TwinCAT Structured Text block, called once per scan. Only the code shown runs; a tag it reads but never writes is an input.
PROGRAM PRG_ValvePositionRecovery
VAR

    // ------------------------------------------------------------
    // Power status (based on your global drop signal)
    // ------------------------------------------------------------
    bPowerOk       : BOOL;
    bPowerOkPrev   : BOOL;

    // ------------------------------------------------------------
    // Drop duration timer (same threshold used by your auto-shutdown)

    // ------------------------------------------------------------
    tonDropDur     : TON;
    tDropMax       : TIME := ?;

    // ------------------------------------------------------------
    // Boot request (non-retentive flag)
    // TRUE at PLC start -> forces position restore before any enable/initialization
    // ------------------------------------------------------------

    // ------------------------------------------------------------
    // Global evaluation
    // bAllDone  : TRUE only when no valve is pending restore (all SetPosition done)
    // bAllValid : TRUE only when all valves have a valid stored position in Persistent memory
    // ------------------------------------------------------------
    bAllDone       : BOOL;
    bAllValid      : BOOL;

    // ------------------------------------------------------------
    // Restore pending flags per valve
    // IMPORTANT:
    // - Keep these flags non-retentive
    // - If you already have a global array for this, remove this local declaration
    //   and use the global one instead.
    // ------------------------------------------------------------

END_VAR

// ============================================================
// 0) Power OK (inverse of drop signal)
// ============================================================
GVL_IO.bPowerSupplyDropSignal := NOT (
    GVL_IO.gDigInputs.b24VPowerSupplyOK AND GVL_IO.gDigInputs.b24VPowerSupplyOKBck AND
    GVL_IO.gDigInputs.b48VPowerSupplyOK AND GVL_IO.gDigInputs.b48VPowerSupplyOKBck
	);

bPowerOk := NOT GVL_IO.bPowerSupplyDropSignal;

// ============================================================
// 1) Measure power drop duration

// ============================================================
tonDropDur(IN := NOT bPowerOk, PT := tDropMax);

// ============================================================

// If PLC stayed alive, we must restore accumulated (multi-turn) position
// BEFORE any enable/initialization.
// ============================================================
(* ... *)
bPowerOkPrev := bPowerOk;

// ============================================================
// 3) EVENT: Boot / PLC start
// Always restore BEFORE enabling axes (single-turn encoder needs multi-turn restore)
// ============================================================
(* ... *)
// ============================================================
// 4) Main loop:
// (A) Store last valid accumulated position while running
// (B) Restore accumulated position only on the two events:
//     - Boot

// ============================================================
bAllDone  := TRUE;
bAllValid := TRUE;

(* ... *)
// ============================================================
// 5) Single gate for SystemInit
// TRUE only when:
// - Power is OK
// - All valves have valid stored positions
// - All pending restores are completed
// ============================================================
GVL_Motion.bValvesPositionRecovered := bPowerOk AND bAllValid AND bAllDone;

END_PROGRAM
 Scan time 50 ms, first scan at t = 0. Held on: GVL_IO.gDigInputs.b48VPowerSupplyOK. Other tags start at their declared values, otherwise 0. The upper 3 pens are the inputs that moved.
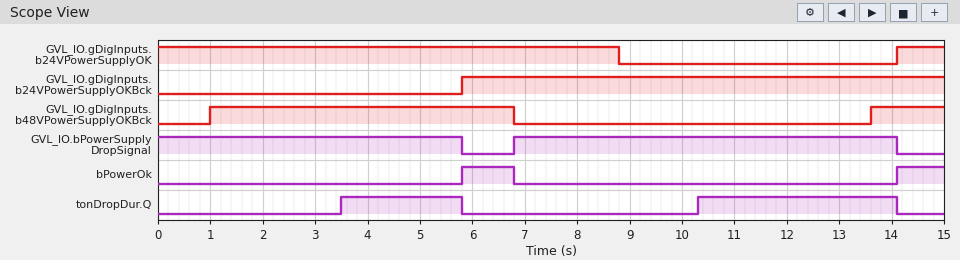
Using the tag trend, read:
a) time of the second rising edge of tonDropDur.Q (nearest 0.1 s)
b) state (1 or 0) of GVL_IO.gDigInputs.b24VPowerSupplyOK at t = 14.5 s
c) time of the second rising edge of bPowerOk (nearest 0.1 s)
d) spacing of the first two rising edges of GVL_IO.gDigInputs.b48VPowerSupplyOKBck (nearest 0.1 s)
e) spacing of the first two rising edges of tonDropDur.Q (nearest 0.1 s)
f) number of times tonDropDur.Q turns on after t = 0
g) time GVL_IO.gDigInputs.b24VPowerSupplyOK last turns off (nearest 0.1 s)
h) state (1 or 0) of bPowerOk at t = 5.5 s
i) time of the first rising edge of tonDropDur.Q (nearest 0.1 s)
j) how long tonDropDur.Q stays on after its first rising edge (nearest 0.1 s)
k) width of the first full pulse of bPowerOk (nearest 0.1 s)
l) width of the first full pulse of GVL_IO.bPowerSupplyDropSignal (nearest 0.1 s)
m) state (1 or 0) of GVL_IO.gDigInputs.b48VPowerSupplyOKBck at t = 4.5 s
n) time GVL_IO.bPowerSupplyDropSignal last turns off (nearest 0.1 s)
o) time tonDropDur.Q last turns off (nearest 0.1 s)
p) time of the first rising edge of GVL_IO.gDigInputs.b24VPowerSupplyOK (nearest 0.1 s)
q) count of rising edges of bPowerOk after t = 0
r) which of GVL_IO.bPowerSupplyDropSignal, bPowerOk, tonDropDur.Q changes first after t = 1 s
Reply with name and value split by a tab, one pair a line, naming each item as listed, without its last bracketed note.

time of the second rising edge of tonDropDur.Q	10.3 s
state (1 or 0) of GVL_IO.gDigInputs.b24VPowerSupplyOK at t = 14.5 s	1
time of the second rising edge of bPowerOk	14.1 s
spacing of the first two rising edges of GVL_IO.gDigInputs.b48VPowerSupplyOKBck	12.6 s
spacing of the first two rising edges of tonDropDur.Q	6.8 s
number of times tonDropDur.Q turns on after t = 0	2
time GVL_IO.gDigInputs.b24VPowerSupplyOK last turns off	8.8 s
state (1 or 0) of bPowerOk at t = 5.5 s	0
time of the first rising edge of tonDropDur.Q	3.5 s
how long tonDropDur.Q stays on after its first rising edge	2.3 s
width of the first full pulse of bPowerOk	1.0 s
width of the first full pulse of GVL_IO.bPowerSupplyDropSignal	7.3 s
state (1 or 0) of GVL_IO.gDigInputs.b48VPowerSupplyOKBck at t = 4.5 s	1
time GVL_IO.bPowerSupplyDropSignal last turns off	14.1 s
time tonDropDur.Q last turns off	14.1 s
time of the first rising edge of GVL_IO.gDigInputs.b24VPowerSupplyOK	14.1 s
count of rising edges of bPowerOk after t = 0	2
which of GVL_IO.bPowerSupplyDropSignal, bPowerOk, tonDropDur.Q changes first after t = 1 s	tonDropDur.Q
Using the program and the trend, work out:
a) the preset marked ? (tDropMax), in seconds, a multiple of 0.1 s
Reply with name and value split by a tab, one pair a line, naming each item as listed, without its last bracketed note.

the preset marked ? (tDropMax), in seconds, a multiple of 0.1 s	3.5 s
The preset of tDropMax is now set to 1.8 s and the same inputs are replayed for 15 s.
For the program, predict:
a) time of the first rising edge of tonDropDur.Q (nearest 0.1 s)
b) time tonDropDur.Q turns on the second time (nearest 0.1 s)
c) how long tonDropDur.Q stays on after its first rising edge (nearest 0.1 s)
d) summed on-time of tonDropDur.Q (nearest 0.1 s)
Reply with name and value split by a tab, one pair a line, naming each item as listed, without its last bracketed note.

time of the first rising edge of tonDropDur.Q	1.8 s
time tonDropDur.Q turns on the second time	8.6 s
how long tonDropDur.Q stays on after its first rising edge	4.0 s
summed on-time of tonDropDur.Q	9.5 s
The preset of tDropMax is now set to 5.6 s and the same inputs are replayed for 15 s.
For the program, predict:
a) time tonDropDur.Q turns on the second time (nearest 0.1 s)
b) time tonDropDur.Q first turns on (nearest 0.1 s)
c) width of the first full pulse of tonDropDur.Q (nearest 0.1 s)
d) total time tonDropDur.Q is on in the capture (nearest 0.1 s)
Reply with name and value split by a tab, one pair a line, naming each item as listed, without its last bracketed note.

time tonDropDur.Q turns on the second time	12.4 s
time tonDropDur.Q first turns on	5.6 s
width of the first full pulse of tonDropDur.Q	0.2 s
total time tonDropDur.Q is on in the capture	1.9 s
